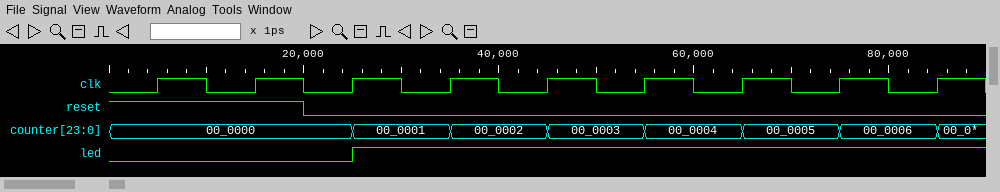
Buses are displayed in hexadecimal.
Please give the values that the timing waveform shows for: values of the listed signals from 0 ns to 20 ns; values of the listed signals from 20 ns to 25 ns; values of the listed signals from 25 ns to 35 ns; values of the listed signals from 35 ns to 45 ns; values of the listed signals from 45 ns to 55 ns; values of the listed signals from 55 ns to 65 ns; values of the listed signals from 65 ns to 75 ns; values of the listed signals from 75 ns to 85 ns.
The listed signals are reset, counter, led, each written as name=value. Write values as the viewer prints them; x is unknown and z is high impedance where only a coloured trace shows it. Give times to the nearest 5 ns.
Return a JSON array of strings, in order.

["reset=1, counter=00_0000, led=0", "reset=0, counter=00_0000, led=0", "reset=0, counter=00_0001, led=1", "reset=0, counter=00_0002, led=1", "reset=0, counter=00_0003, led=1", "reset=0, counter=00_0004, led=1", "reset=0, counter=00_0005, led=1", "reset=0, counter=00_0006, led=1"]
